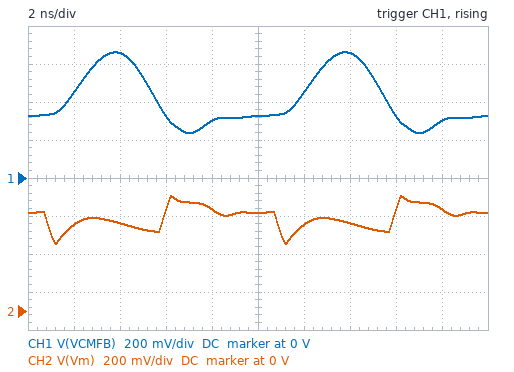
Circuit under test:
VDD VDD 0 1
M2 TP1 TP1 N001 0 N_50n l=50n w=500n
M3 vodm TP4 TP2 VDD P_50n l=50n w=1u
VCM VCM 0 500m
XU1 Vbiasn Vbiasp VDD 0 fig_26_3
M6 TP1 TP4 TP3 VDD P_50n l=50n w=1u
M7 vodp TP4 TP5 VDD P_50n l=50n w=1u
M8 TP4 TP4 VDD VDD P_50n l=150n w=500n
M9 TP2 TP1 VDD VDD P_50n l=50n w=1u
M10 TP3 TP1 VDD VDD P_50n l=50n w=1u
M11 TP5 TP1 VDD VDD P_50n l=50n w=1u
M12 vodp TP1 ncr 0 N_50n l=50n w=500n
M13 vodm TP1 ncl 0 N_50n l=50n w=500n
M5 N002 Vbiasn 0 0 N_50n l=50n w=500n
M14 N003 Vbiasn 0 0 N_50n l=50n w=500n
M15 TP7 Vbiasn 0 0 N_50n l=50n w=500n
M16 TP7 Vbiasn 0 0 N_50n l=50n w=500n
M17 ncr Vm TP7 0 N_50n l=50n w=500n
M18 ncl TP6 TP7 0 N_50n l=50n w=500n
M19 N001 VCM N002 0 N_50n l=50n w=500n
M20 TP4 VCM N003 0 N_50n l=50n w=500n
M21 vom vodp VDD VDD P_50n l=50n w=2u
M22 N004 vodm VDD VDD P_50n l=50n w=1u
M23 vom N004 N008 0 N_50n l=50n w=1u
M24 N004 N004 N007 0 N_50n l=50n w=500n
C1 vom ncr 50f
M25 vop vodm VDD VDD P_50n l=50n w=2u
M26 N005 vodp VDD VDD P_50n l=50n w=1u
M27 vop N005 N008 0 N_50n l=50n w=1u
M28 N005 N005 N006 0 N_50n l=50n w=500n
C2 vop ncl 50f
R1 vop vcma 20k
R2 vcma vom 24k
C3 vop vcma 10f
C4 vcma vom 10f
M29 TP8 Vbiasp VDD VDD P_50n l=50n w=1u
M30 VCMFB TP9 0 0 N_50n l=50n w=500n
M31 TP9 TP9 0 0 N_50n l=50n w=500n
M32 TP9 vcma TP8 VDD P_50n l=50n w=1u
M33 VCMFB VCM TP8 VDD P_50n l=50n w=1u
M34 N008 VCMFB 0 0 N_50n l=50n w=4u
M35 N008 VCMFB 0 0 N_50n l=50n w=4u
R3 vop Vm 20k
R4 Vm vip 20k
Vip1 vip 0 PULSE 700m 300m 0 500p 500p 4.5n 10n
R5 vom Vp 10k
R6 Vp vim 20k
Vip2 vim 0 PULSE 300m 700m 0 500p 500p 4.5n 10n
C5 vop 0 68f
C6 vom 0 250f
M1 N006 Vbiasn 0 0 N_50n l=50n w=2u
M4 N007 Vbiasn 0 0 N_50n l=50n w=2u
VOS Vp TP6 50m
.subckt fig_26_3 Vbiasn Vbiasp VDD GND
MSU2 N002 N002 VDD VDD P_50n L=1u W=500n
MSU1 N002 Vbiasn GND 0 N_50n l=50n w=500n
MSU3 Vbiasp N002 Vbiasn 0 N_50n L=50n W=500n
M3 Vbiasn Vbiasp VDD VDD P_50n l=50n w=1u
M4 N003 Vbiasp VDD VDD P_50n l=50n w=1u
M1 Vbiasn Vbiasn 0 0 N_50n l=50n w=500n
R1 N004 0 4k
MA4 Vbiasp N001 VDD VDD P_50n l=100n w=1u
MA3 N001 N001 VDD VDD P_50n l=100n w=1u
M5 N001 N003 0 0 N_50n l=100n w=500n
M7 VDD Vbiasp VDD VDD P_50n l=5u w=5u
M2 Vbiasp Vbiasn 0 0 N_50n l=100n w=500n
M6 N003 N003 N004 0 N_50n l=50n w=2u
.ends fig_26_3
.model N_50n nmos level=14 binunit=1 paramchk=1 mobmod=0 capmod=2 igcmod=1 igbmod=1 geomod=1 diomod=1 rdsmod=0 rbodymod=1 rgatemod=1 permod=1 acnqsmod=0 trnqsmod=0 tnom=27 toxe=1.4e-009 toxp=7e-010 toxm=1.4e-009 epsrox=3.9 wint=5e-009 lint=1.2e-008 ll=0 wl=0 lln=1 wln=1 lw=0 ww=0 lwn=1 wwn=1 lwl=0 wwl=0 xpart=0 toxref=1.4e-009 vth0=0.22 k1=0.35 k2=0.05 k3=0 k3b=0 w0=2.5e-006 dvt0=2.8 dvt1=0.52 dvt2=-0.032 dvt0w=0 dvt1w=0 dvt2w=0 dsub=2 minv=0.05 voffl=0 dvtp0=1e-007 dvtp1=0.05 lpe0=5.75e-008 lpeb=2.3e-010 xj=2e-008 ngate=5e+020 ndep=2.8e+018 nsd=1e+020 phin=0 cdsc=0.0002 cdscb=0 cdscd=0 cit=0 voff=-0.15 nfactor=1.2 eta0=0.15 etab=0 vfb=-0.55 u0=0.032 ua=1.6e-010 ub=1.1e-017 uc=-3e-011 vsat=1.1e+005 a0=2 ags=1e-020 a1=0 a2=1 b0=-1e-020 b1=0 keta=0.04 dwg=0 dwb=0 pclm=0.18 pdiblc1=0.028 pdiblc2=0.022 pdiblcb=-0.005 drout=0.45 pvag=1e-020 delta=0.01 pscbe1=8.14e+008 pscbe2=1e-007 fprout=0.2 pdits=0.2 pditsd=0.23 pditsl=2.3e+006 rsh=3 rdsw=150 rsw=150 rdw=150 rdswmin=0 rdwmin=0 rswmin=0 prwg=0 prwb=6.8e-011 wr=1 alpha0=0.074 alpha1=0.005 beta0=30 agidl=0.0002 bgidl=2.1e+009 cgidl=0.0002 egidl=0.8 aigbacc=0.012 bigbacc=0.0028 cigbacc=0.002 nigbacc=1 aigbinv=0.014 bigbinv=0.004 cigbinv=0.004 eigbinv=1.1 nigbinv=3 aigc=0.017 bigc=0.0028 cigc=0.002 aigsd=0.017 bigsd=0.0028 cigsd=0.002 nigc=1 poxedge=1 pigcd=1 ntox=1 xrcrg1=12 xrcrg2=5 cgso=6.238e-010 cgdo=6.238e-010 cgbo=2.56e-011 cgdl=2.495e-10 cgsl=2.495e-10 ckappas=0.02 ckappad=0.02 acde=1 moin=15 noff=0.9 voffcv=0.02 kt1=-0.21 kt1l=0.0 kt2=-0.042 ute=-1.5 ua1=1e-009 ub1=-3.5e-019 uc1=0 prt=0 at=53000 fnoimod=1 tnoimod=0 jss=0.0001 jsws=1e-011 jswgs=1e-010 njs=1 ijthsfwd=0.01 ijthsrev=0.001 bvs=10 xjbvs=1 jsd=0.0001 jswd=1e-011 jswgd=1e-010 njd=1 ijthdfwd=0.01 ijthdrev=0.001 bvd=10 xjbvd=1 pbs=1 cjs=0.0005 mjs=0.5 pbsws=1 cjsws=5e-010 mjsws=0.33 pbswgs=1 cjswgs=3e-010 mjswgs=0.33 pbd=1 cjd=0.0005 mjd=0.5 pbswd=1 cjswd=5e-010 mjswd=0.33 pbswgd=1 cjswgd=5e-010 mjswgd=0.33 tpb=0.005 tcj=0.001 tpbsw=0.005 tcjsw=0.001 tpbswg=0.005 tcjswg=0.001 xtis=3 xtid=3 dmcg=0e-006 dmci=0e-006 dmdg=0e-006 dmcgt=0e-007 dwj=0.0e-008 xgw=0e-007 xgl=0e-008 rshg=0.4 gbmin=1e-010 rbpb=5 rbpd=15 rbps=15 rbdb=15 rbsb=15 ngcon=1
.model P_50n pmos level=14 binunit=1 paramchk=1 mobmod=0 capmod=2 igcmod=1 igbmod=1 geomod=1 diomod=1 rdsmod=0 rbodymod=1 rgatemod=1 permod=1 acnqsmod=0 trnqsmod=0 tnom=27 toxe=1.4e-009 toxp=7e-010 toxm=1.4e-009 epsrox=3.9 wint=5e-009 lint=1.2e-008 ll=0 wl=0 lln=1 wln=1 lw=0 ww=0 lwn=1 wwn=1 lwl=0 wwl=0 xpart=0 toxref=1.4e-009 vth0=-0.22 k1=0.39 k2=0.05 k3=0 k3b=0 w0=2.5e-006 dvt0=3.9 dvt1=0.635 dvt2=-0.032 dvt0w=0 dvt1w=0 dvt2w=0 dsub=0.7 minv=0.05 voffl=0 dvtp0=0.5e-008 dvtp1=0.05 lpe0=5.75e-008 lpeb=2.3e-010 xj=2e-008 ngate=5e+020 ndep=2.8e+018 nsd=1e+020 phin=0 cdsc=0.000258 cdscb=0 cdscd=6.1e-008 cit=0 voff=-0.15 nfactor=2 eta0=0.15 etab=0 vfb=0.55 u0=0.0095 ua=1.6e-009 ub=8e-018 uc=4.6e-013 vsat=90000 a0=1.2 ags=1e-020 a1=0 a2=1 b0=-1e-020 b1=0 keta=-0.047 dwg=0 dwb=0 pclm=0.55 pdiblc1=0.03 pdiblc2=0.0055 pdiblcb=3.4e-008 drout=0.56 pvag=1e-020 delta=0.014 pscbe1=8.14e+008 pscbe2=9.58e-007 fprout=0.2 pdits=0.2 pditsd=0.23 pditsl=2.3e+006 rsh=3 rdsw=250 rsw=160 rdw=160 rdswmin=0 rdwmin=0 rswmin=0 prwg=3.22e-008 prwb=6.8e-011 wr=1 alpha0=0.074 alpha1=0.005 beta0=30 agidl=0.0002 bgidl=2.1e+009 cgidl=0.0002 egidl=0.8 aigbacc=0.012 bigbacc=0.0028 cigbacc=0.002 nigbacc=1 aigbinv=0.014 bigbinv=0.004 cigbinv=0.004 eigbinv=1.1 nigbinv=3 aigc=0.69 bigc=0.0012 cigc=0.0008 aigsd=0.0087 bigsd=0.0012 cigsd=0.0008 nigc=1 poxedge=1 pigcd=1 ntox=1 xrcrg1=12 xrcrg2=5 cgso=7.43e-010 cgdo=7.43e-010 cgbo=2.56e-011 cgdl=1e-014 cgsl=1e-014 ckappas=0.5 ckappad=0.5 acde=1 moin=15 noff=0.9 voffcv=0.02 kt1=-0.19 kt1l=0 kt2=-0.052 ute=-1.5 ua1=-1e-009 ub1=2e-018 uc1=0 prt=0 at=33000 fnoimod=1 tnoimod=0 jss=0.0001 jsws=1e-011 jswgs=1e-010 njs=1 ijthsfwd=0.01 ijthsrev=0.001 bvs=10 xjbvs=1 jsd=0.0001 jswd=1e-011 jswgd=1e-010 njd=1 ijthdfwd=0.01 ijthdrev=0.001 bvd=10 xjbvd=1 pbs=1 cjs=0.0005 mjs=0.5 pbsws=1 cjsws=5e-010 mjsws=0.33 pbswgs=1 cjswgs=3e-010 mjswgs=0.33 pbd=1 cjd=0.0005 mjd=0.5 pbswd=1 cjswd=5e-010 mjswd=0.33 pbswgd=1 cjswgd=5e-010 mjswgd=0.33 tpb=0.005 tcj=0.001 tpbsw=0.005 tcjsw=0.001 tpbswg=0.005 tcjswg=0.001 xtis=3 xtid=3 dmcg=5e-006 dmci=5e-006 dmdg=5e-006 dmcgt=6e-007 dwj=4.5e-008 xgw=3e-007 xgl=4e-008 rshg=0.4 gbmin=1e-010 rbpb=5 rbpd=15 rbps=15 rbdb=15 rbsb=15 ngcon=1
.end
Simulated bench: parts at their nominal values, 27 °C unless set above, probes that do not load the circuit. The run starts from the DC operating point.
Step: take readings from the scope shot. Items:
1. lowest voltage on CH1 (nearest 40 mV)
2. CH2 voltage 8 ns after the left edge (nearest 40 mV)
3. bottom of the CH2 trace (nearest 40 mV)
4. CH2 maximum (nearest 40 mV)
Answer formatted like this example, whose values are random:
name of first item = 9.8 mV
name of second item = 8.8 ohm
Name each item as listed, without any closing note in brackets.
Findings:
lowest voltage on CH1 = 240 mV
CH2 voltage 8 ns after the left edge = 520 mV
bottom of the CH2 trace = 360 mV
CH2 maximum = 600 mV
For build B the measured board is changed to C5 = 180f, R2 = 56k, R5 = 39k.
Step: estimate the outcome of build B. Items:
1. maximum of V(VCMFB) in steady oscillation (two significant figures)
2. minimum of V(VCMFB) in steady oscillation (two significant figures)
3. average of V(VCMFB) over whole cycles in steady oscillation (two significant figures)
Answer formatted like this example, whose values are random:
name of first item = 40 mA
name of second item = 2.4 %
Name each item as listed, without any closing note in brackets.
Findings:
maximum of V(VCMFB) in steady oscillation = 790 mV
minimum of V(VCMFB) in steady oscillation = 230 mV
average of V(VCMFB) over whole cycles in steady oscillation = 440 mV
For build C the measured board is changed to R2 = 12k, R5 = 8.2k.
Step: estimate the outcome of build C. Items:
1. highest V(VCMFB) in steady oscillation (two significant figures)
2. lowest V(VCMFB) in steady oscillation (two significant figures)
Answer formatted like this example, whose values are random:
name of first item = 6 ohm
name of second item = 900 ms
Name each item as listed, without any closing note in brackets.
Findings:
highest V(VCMFB) in steady oscillation = 430 mV
lowest V(VCMFB) in steady oscillation = 260 mV
